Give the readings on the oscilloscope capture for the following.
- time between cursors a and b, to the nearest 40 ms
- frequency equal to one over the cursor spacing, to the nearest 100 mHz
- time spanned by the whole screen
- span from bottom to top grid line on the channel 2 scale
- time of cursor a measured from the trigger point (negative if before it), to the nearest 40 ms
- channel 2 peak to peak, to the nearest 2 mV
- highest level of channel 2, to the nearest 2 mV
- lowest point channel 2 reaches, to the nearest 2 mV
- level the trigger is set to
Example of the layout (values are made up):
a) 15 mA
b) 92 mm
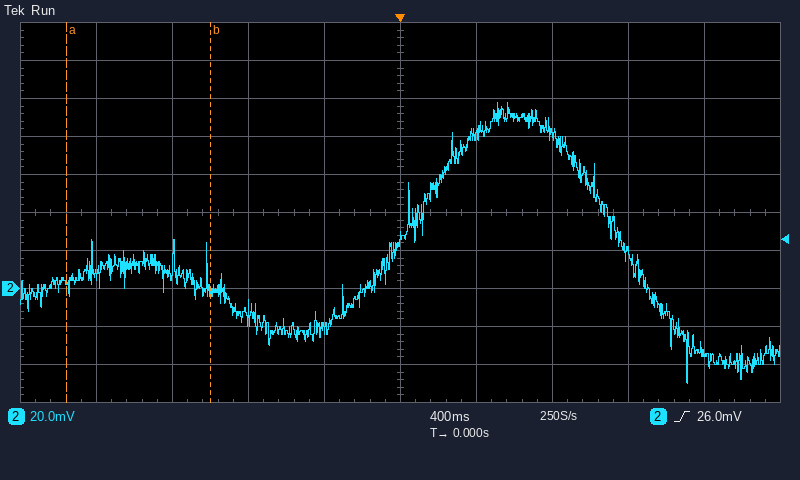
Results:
a) 760 ms
b) 1.3 Hz
c) 4 s
d) 200 mV
e) -1.76 s
f) 148 mV
g) 98 mV
h) -50 mV
i) 26.0 mV
